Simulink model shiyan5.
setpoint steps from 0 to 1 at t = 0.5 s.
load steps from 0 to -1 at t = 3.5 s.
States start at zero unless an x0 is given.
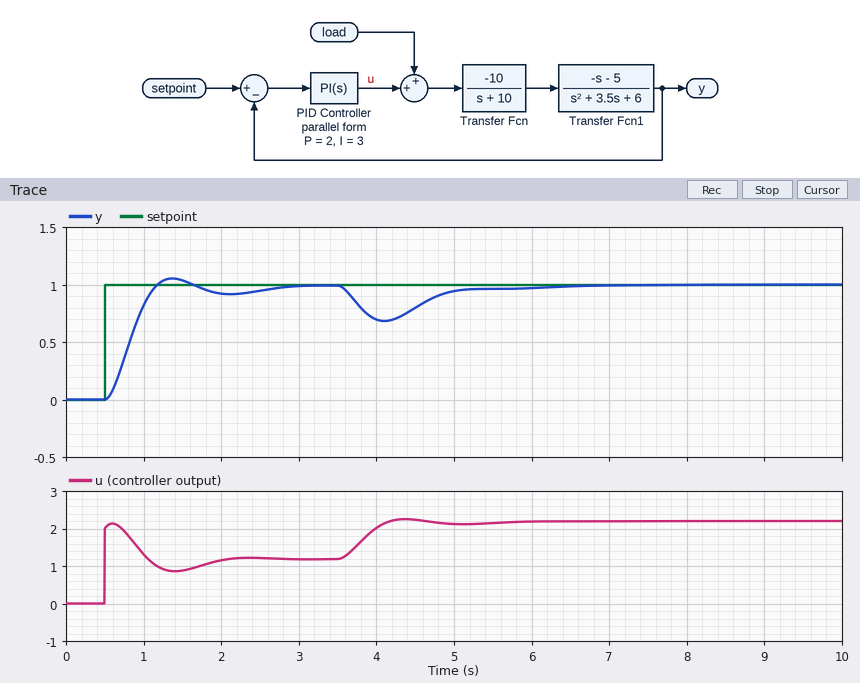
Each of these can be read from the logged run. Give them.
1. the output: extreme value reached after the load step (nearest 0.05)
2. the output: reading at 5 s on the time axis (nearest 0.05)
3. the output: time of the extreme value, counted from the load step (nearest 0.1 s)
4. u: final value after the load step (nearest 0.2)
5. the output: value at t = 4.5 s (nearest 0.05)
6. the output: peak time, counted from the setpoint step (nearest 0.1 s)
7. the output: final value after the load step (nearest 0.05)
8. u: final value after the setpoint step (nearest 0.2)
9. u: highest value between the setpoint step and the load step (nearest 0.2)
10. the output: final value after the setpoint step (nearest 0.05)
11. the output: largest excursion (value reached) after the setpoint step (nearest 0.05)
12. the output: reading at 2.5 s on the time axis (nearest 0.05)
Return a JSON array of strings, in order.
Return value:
["0.70", "0.95", "0.6 s", "2.2", "0.80", "0.9 s", "1.00", "1.2", "2.2", "1.00", "1.05", "0.95"]
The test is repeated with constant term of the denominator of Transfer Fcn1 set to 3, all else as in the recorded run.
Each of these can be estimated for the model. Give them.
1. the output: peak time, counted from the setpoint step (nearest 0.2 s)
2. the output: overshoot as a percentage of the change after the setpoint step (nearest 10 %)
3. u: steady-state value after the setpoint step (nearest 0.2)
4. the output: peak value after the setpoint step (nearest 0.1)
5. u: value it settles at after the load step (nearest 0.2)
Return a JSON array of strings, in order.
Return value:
["1.0 s", "20 %", "0.6", "1.2", "1.6"]
